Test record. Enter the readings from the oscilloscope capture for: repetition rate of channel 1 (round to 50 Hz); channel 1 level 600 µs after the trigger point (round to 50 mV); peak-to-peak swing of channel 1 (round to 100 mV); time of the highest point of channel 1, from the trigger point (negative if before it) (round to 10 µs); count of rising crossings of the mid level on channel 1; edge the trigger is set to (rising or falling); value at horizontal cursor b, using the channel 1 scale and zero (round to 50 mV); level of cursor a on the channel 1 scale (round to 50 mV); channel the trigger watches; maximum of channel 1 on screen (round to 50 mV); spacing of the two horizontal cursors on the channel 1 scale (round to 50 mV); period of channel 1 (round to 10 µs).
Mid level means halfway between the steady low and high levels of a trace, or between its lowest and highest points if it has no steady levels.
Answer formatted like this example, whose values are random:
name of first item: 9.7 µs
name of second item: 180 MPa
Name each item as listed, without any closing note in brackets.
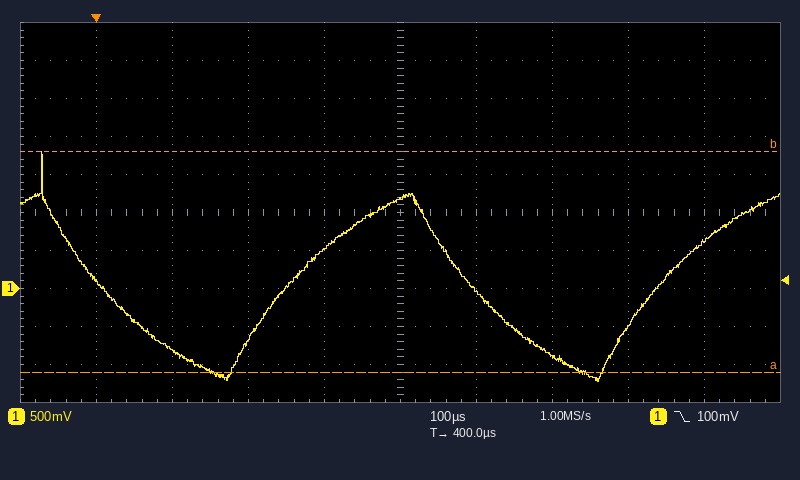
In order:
repetition rate of channel 1: 2.05 kHz
channel 1 level 600 µs after the trigger point: -900 mV
peak-to-peak swing of channel 1: 3.00 V
time of the highest point of channel 1, from the trigger point (negative if before it): -70 µs
count of rising crossings of the mid level on channel 1: 2
edge the trigger is set to: falling
value at horizontal cursor b, using the channel 1 scale and zero: 1.80 V
level of cursor a on the channel 1 scale: -1.10 V
channel the trigger watches: channel 1
maximum of channel 1 on screen: 1.80 V
spacing of the two horizontal cursors on the channel 1 scale: 2.90 V
period of channel 1: 490 µs
